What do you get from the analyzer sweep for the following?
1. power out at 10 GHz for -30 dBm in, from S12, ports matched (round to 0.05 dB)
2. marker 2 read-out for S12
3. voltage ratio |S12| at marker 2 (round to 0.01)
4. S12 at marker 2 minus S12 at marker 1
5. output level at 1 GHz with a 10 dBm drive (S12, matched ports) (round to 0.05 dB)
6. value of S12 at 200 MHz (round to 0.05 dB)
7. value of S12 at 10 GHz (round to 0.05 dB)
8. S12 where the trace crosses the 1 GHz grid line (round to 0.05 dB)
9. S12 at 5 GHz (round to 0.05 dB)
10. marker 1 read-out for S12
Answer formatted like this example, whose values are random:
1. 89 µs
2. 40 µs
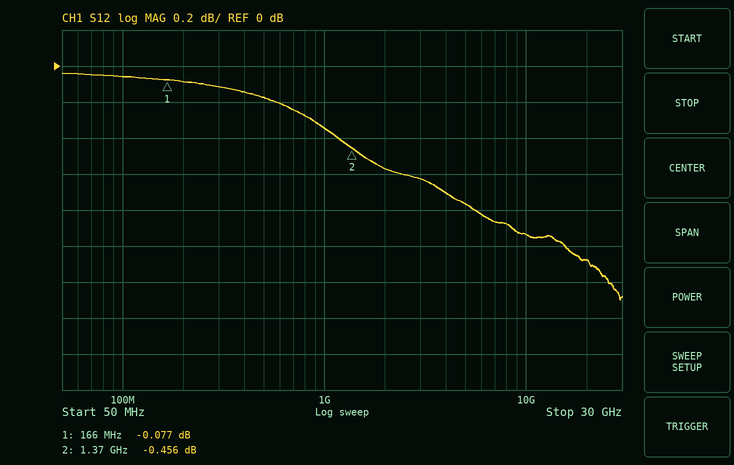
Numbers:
1. -30.95 dBm
2. -0.456 dB
3. 0.95
4. -0.379 dB
5. 9.65 dBm
6. -0.10 dB
7. -0.95 dB
8. -0.35 dB
9. -0.75 dB
10. -0.077 dB
